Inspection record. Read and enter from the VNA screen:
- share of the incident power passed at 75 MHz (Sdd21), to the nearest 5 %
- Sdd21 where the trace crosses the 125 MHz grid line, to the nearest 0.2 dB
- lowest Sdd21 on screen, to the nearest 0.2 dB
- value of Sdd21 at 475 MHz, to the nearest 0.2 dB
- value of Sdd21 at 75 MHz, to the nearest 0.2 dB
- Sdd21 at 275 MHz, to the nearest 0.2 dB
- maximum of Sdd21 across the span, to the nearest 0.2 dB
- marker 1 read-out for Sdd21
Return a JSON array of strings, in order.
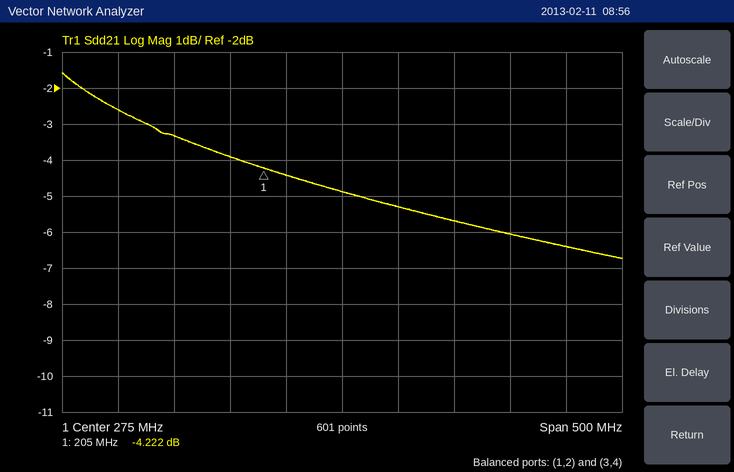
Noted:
["55 %", "-3.4 dB", "-6.8 dB", "-6.4 dB", "-2.6 dB", "-4.8 dB", "-1.6 dB", "-4.222 dB"]
